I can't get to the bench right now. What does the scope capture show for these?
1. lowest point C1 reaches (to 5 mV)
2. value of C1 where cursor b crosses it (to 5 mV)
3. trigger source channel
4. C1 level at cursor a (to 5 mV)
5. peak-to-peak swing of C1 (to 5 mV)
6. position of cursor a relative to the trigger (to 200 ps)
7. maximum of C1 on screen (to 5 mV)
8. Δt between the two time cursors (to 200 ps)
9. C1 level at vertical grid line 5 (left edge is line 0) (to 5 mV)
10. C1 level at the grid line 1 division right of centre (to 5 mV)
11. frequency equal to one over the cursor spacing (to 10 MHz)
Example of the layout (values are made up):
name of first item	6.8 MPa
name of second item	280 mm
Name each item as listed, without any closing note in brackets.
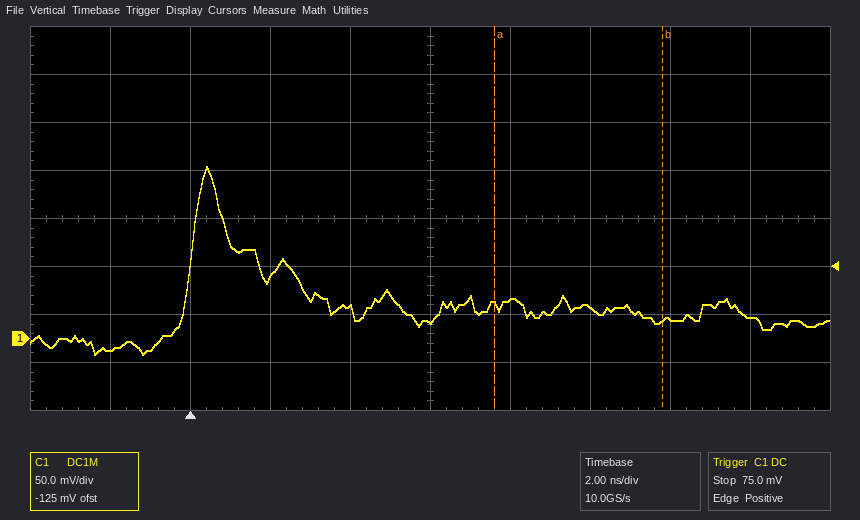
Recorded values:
lowest point C1 reaches	-15 mV
value of C1 where cursor b crosses it	20 mV
trigger source channel	C1
C1 level at cursor a	35 mV
peak-to-peak swing of C1	195 mV
position of cursor a relative to the trigger	+7.6 ns
maximum of C1 on screen	180 mV
Δt between the two time cursors	4.2 ns
C1 level at vertical grid line 5 (left edge is line 0)	20 mV
C1 level at the grid line 1 division right of centre	40 mV
frequency equal to one over the cursor spacing	240 MHz
